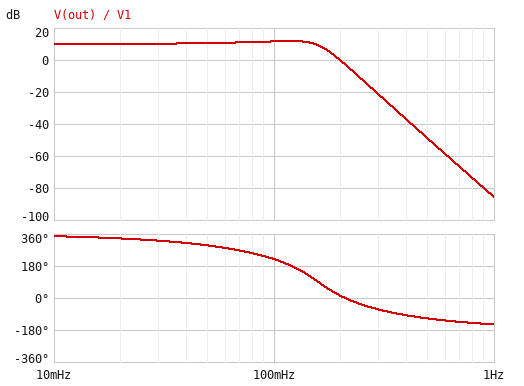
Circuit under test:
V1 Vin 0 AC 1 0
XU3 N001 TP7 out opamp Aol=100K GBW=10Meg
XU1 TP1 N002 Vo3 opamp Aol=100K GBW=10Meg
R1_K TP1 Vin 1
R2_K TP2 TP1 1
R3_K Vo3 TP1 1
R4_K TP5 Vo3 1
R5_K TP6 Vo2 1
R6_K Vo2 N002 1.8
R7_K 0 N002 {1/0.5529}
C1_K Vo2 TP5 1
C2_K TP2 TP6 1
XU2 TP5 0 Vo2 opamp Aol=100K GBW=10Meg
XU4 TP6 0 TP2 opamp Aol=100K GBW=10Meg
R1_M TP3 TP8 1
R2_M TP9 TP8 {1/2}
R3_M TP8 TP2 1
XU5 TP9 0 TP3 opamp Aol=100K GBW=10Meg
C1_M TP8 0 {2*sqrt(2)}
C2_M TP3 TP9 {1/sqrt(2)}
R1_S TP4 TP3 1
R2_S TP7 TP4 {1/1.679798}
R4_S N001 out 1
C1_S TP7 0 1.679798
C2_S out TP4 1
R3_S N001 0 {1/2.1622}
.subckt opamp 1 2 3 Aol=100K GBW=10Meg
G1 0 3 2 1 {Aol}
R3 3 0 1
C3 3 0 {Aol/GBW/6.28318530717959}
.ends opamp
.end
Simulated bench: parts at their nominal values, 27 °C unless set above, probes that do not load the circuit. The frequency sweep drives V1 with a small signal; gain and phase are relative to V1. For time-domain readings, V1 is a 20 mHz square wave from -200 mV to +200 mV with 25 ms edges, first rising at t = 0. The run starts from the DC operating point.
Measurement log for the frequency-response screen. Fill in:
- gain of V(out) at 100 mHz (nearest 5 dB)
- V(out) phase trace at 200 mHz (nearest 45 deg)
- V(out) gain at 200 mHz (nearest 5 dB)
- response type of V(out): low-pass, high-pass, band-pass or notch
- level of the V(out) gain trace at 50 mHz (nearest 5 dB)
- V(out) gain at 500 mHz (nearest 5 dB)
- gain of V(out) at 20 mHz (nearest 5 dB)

10 dB
0 deg
0 dB
low-pass
10 dB
-50 dB
10 dB
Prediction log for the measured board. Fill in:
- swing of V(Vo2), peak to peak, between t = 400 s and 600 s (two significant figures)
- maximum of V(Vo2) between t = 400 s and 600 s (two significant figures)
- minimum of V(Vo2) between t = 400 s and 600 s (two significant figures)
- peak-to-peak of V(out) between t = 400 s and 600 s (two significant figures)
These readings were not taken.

350 mV
180 mV
-180 mV
1.9 V
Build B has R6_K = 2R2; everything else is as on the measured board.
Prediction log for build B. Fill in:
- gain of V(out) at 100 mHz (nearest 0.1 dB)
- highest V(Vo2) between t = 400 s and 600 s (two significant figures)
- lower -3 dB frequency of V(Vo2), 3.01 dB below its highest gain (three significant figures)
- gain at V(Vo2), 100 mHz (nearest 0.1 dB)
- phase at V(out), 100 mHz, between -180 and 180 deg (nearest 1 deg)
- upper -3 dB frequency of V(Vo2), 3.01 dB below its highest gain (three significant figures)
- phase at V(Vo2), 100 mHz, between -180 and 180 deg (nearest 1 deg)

12.3 dB
190 mV
84.5 mHz
-4.4 dB
-139 deg
300 mHz
35 deg
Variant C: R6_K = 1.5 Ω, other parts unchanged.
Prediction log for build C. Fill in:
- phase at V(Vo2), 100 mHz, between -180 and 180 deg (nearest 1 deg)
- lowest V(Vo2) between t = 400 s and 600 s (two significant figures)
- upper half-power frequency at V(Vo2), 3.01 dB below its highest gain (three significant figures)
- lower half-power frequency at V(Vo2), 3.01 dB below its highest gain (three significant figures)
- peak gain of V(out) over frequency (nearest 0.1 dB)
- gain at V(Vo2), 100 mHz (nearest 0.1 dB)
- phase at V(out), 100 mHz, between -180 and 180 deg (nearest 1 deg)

30 deg
-170 mV
336 mHz
75.3 mHz
11.2 dB
-5.6 dB
-144 deg
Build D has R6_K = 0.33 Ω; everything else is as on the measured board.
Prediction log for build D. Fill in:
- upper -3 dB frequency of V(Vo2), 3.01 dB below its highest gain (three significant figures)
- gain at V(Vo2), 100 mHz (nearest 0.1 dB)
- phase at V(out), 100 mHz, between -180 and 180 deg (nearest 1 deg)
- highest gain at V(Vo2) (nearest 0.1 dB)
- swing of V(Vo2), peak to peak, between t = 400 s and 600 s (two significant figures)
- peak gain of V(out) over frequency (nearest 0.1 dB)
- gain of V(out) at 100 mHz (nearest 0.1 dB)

459 mHz
-8.7 dB
-153 deg
-8.1 dB
250 mV
10.0 dB
8.0 dB
